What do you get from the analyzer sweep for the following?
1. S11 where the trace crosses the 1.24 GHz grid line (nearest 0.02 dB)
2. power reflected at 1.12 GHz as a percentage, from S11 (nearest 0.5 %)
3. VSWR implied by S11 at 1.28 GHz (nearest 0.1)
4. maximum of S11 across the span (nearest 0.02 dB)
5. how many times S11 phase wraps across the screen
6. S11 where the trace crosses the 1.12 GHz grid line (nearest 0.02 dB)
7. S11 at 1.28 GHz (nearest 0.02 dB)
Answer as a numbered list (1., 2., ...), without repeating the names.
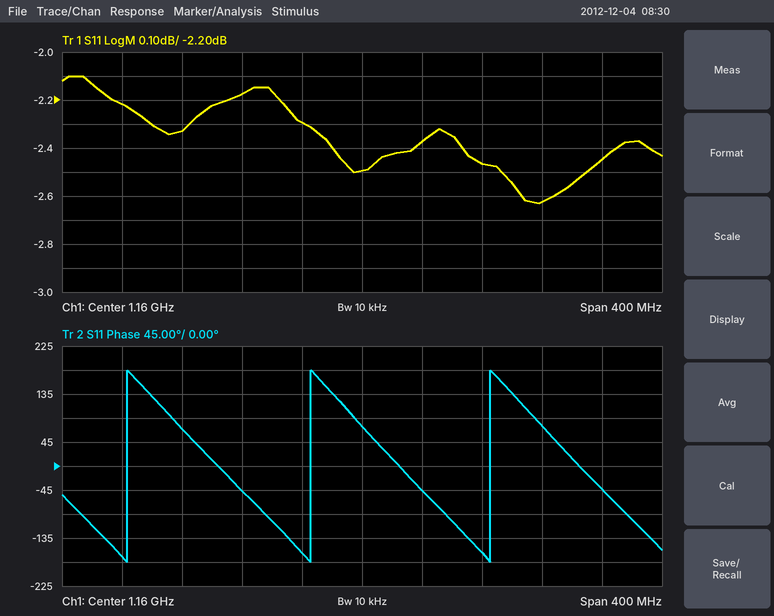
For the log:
1. -2.46 dB
2. 59.0 %
3. 6.7
4. -2.10 dB
5. 3
6. -2.30 dB
7. -2.62 dB
